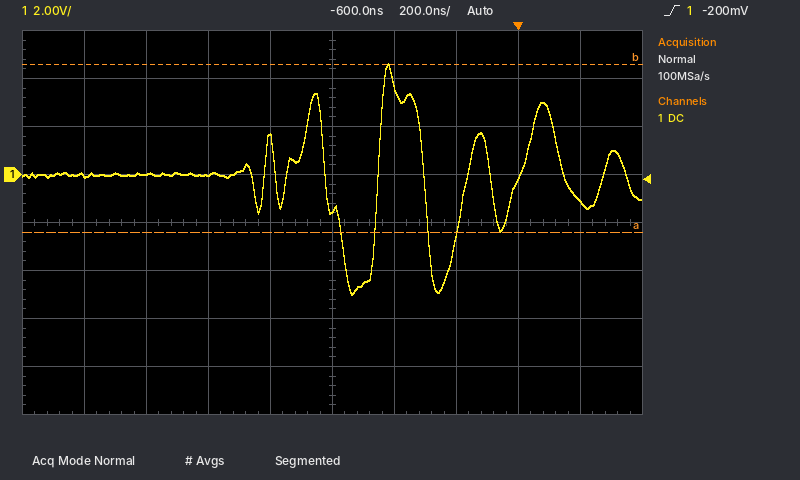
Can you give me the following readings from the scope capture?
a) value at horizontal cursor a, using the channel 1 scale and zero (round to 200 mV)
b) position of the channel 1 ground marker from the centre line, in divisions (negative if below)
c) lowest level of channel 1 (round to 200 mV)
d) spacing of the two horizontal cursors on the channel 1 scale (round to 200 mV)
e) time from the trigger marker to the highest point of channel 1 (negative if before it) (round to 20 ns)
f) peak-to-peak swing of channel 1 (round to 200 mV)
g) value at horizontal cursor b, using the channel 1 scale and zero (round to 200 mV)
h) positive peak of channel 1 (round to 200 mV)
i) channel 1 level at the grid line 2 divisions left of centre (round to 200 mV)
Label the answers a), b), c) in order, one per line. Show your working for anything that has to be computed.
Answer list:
a) -2.4 V
b) +1.0 div
c) -5.0 V
d) 7.0 V
e) -420 ns
f) 4.6 V − (-5.0 V) = 9.6 V
g) 4.6 V
h) 4.6 V
i) 0.0 V
